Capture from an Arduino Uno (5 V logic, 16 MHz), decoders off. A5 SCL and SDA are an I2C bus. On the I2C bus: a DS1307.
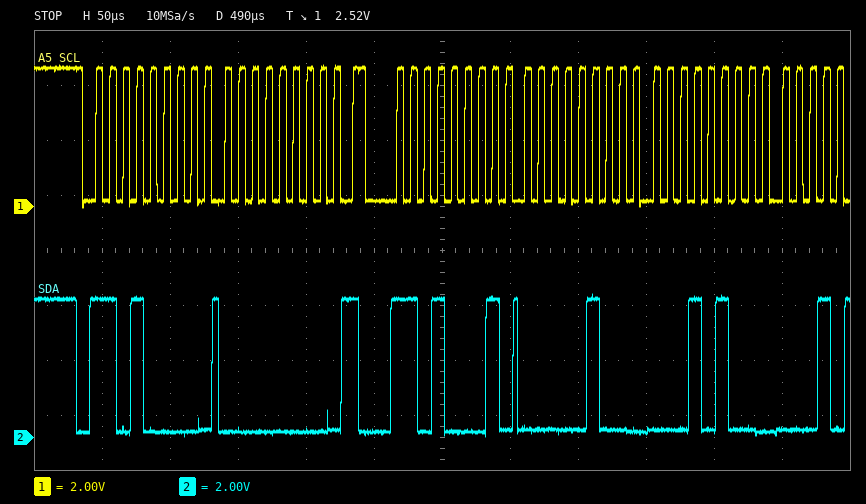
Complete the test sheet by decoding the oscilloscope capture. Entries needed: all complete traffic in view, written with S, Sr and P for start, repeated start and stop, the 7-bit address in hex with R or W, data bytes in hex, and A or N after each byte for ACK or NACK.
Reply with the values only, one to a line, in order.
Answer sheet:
S 68W A 00 A Sr 68R A 04 A 14 A
